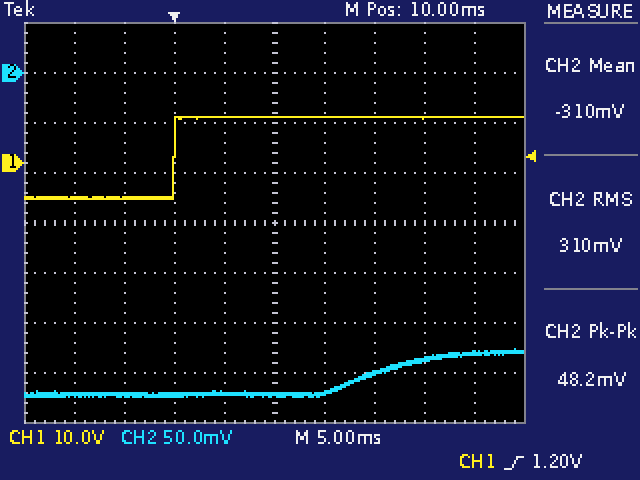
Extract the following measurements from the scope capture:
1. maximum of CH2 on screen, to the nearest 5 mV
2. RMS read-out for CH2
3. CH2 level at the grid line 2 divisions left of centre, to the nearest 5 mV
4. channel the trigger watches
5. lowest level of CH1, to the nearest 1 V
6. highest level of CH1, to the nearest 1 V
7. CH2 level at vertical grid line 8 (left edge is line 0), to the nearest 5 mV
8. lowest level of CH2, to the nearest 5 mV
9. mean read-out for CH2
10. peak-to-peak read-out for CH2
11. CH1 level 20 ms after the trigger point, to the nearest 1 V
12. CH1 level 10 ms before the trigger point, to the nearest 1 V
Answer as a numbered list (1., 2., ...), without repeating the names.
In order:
1. -275 mV
2. 310 mV
3. -320 mV
4. CH1
5. -7 V
6. 9 V
7. -285 mV
8. -325 mV
9. -310 mV
10. 48.2 mV
11. 9 V
12. -7 V
